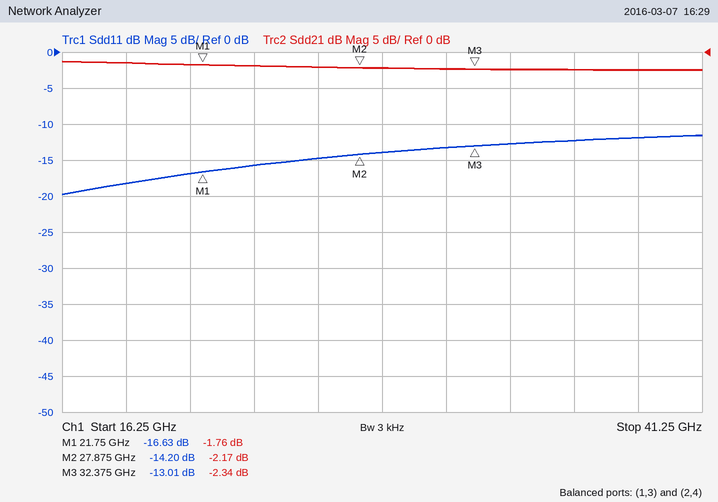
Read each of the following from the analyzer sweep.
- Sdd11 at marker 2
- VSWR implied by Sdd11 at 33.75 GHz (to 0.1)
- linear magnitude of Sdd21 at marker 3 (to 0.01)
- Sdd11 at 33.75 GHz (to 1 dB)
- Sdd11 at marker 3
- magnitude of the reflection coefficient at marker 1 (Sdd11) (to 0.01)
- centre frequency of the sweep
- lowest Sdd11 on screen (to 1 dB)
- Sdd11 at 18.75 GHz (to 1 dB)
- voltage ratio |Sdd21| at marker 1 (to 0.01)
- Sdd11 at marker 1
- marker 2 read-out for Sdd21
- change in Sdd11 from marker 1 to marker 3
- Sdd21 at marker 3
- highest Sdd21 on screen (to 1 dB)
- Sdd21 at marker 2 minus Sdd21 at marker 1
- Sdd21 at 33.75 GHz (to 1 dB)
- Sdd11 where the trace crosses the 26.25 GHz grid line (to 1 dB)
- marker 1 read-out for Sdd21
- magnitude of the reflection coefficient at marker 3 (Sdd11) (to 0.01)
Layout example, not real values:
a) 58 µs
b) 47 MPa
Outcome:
a) -14.20 dB
b) 1.6
c) 0.76
d) -13 dB
e) -13.01 dB
f) 0.15
g) 28.75 GHz
h) -20 dB
i) -18 dB
j) 0.82
k) -16.63 dB
l) -2.17 dB
m) 3.62 dB
n) -2.34 dB
o) -1 dB
p) -0.41 dB
q) -2 dB
r) -15 dB
s) -1.76 dB
t) 0.22
